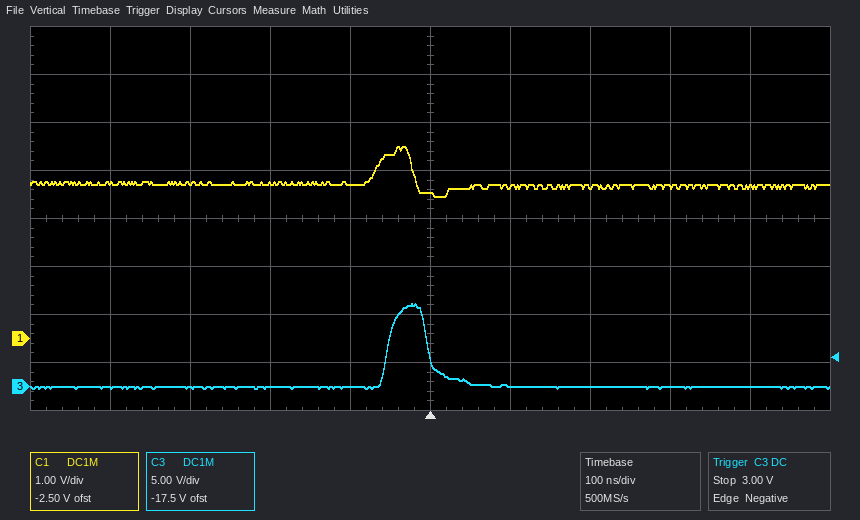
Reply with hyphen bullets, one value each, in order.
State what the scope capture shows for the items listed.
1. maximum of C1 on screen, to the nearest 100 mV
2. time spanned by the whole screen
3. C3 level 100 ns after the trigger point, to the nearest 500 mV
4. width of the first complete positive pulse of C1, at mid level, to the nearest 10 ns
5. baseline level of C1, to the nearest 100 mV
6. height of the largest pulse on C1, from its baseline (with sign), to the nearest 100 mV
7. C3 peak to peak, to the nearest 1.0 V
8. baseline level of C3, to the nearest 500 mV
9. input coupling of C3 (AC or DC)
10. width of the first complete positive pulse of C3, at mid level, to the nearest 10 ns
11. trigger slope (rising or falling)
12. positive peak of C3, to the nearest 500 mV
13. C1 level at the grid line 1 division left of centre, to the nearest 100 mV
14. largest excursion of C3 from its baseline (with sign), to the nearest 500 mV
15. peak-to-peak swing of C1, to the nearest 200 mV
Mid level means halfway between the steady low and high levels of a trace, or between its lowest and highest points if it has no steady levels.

- 4.0 V
- 1 µs
- 0.0 V
- 50 ns
- 3.2 V
- +800 mV
- 9.0 V
- 0.0 V
- DC
- 50 ns
- falling
- 8.5 V
- 3.2 V
- +8.5 V
- 1.0 V
